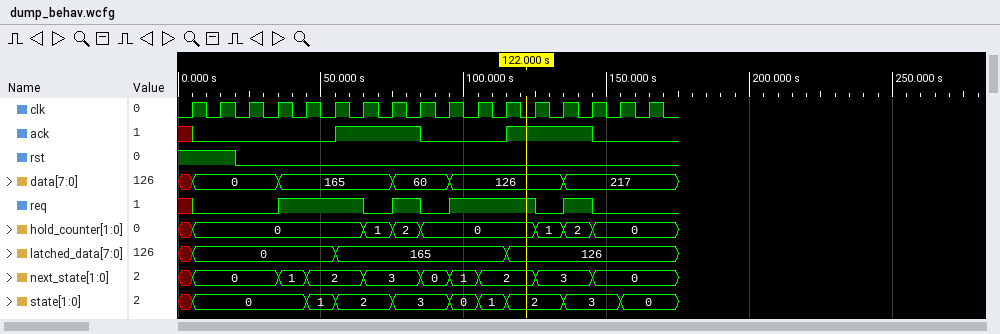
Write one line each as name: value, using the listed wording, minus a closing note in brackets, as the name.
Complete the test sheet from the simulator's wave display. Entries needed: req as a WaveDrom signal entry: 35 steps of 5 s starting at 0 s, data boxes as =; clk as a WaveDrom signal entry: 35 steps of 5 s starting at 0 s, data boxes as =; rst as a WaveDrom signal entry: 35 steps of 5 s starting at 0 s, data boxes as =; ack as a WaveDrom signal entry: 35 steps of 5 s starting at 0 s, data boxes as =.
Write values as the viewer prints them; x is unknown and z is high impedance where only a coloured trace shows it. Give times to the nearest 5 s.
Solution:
req as a WaveDrom signal entry: 35 steps of 5 s starting at 0 s, data boxes as =: {name: 'req', wave: 'x0.....1.....0.1.0.1.....0.1.0.....'}
clk as a WaveDrom signal entry: 35 steps of 5 s starting at 0 s, data boxes as =: {name: 'clk', wave: '01010101010101010101010101010101010'}
rst as a WaveDrom signal entry: 35 steps of 5 s starting at 0 s, data boxes as =: {name: 'rst', wave: '1...0..............................'}
ack as a WaveDrom signal entry: 35 steps of 5 s starting at 0 s, data boxes as =: {name: 'ack', wave: 'x0.........1.....0.....1.....0.....'}
